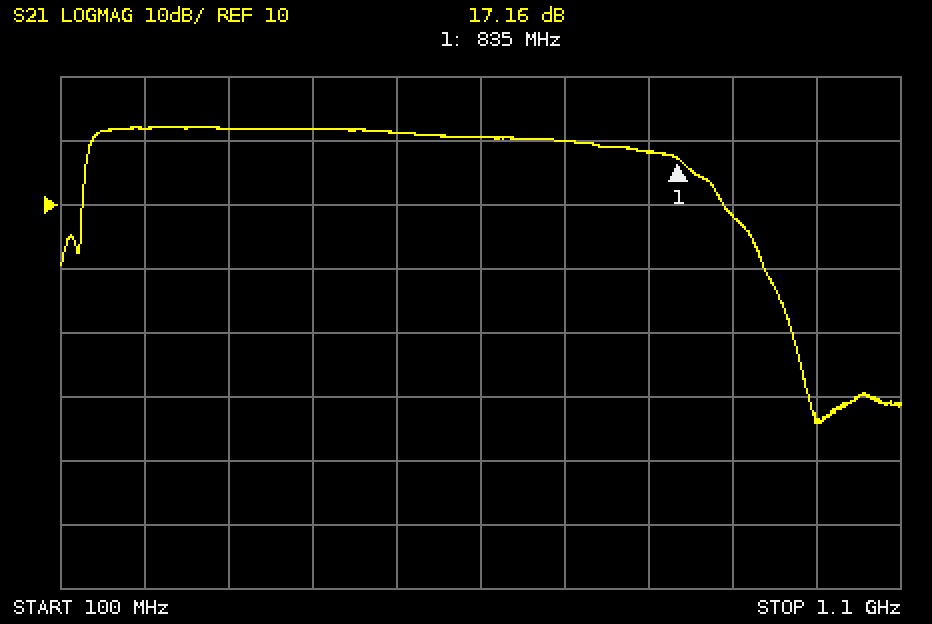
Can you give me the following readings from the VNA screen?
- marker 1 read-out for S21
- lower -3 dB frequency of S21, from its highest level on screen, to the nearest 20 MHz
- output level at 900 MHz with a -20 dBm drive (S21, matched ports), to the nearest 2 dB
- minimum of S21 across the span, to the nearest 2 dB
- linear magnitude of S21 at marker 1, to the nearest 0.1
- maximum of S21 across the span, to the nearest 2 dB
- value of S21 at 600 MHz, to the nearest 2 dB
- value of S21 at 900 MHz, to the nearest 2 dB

17.16 dB
140 MHz
-12 dBm
-24 dB
7.2
22 dB
20 dB
8 dB
